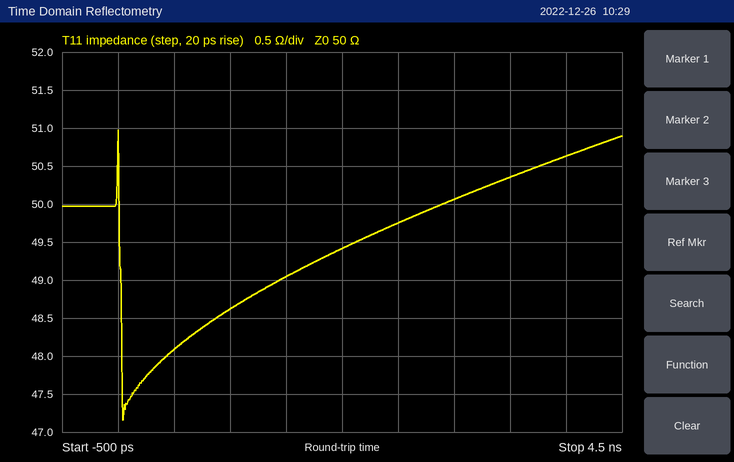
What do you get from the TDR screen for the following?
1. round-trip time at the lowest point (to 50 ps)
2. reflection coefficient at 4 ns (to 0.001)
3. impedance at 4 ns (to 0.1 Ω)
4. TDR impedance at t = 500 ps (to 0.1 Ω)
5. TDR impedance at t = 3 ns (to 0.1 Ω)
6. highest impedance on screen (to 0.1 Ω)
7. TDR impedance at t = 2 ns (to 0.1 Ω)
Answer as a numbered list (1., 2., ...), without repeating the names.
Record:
1. 50 ps
2. +0.006
3. 50.6 Ω
4. 48.1 Ω
5. 50.1 Ω
6. 51.0 Ω
7. 49.4 Ω
